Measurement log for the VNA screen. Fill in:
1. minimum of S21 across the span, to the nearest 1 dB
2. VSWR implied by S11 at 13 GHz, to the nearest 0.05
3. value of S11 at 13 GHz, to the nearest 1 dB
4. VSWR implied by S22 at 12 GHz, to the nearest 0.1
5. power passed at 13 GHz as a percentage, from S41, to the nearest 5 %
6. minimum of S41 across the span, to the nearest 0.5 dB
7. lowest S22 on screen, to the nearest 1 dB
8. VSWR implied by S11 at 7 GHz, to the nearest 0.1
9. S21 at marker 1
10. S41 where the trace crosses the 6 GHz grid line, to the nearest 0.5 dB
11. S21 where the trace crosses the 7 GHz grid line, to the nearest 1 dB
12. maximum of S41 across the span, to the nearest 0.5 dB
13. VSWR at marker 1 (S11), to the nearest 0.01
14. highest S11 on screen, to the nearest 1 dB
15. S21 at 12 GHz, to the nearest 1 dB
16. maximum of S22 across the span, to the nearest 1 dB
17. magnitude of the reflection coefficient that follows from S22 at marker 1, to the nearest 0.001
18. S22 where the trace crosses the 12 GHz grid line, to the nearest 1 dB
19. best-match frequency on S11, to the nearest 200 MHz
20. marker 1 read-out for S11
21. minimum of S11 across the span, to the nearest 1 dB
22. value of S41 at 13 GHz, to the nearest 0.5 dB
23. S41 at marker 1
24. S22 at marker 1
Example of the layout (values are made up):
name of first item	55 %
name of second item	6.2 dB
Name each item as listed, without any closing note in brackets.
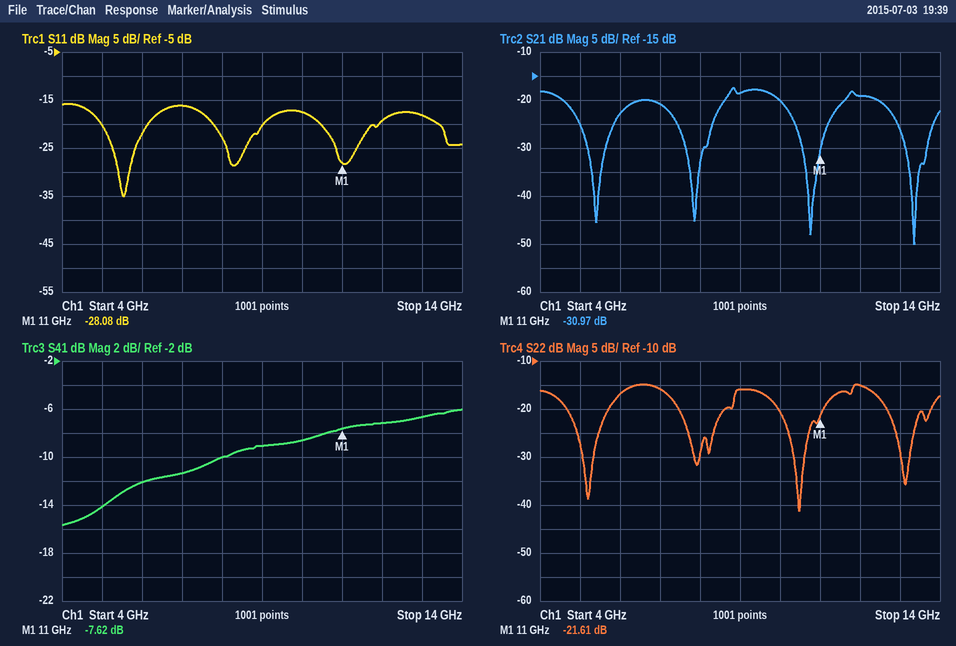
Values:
minimum of S21 across the span, to the nearest 1 dB	-50 dB
VSWR implied by S11 at 13 GHz, to the nearest 0.05	1.30
value of S11 at 13 GHz, to the nearest 1 dB	-18 dB
VSWR implied by S22 at 12 GHz, to the nearest 0.1	1.4
power passed at 13 GHz as a percentage, from S41, to the nearest 5 %	20 %
minimum of S41 across the span, to the nearest 0.5 dB	-15.5 dB
lowest S22 on screen, to the nearest 1 dB	-41 dB
VSWR implied by S11 at 7 GHz, to the nearest 0.1	1.4
S21 at marker 1	-30.97 dB
S41 where the trace crosses the 6 GHz grid line, to the nearest 0.5 dB	-12.0 dB
S21 where the trace crosses the 7 GHz grid line, to the nearest 1 dB	-21 dB
maximum of S41 across the span, to the nearest 0.5 dB	-6.0 dB
VSWR at marker 1 (S11), to the nearest 0.01	1.08
highest S11 on screen, to the nearest 1 dB	-16 dB
S21 at 12 GHz, to the nearest 1 dB	-19 dB
maximum of S22 across the span, to the nearest 1 dB	-15 dB
magnitude of the reflection coefficient that follows from S22 at marker 1, to the nearest 0.001	0.083
S22 where the trace crosses the 12 GHz grid line, to the nearest 1 dB	-15 dB
best-match frequency on S11, to the nearest 200 MHz	5.6 GHz
marker 1 read-out for S11	-28.08 dB
minimum of S11 across the span, to the nearest 1 dB	-35 dB
value of S41 at 13 GHz, to the nearest 0.5 dB	-6.5 dB
S41 at marker 1	-7.62 dB
S22 at marker 1	-21.61 dB
